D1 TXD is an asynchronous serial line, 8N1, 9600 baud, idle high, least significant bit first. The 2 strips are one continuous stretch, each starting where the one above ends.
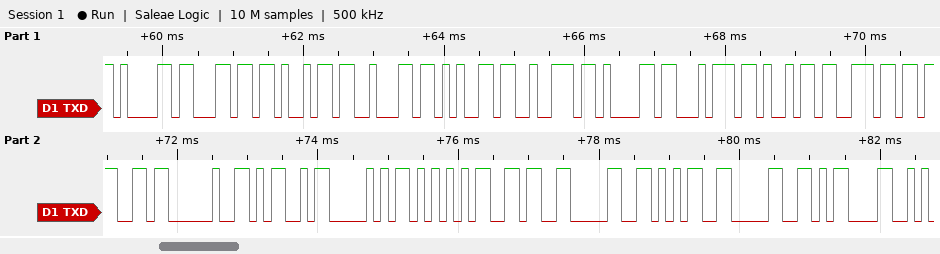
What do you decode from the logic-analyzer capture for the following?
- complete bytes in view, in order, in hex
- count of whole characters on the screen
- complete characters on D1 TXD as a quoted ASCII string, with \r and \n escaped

61 6C 69 62 65 72 61 74 69 6E 67 20 4D 50 55 36 30 35 30 0D
20
"aliberating MPU6050\r"
